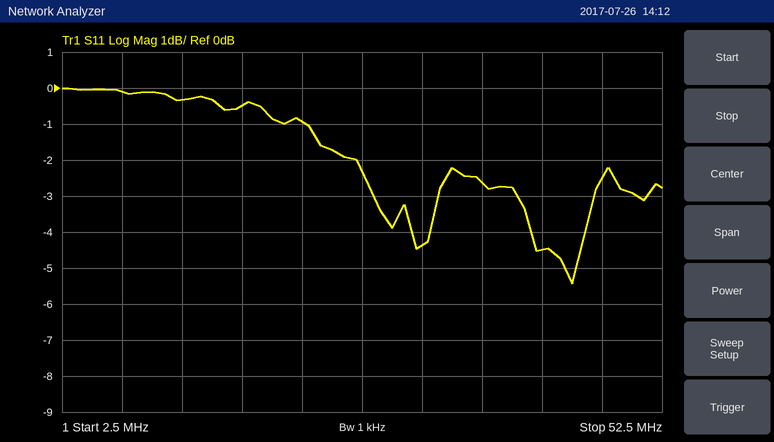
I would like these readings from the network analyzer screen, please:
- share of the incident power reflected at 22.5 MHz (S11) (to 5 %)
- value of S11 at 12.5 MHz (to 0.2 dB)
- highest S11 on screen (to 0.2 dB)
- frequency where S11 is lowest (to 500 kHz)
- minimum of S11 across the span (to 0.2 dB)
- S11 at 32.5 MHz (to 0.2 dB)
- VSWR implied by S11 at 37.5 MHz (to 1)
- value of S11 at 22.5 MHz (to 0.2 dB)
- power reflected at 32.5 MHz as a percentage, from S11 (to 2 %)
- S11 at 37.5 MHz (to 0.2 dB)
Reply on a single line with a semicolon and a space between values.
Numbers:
80 %; -0.4 dB; 0.0 dB; 45.0 MHz; -5.4 dB; -4.4 dB; 7; -1.0 dB; 36 %; -2.6 dB
